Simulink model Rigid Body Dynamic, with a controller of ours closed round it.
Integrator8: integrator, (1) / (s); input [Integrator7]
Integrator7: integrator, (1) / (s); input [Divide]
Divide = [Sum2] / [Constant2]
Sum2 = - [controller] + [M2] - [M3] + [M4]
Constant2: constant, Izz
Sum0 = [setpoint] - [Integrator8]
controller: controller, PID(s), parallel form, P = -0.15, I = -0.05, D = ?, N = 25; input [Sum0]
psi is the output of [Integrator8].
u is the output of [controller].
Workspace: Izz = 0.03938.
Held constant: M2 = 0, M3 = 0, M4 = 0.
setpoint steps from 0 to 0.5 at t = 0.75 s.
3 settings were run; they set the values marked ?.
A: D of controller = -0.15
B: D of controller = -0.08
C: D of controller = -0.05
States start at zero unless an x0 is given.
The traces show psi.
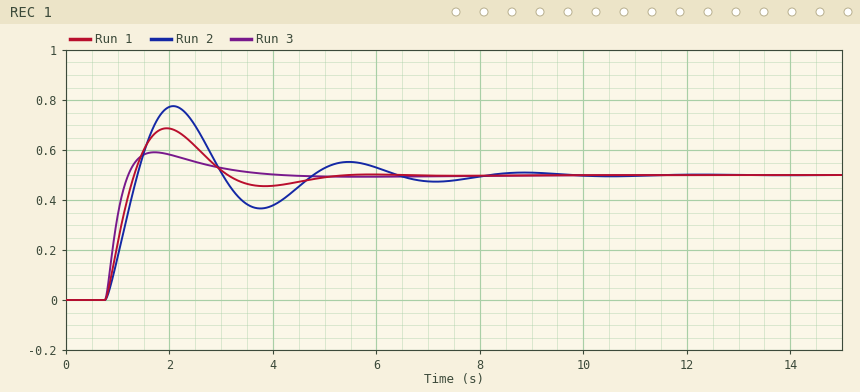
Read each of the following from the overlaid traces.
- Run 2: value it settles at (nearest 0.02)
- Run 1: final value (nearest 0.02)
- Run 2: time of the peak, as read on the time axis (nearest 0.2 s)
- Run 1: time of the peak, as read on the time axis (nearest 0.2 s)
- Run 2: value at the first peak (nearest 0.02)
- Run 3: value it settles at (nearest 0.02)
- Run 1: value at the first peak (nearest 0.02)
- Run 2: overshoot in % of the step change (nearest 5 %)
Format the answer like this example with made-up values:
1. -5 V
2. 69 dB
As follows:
1. 0.50
2. 0.50
3. 2.0 s
4. 2.0 s
5. 0.78
6. 0.50
7. 0.68
8. 55 %
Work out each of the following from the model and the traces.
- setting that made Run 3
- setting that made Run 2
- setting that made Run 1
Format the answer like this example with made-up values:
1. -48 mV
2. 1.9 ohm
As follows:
1. A
2. C
3. B
